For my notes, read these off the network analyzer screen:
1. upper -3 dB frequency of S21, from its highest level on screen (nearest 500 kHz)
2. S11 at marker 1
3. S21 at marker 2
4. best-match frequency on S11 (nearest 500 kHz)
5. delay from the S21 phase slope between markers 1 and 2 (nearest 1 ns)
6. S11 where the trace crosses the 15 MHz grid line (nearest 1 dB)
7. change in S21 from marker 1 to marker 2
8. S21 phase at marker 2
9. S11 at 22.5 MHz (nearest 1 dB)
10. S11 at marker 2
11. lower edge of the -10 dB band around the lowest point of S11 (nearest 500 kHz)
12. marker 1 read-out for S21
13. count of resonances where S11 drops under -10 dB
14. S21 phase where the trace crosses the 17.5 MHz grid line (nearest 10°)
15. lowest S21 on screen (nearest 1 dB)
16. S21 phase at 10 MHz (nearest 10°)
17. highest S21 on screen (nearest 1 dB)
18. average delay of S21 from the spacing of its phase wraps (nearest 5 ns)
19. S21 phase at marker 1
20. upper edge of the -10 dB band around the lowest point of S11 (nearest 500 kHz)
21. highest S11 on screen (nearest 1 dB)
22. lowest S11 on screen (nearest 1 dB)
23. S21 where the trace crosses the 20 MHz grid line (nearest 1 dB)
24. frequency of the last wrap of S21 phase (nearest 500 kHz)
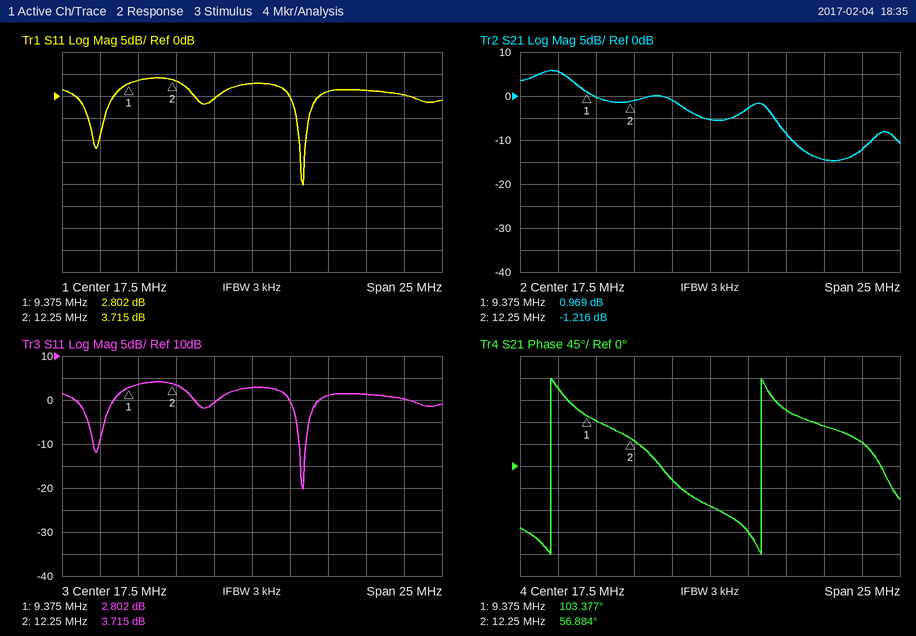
8.5 MHz
2.802 dB
-1.216 dB
21.0 MHz
45 ns
-1 dB
-2.185 dB
56.884°
1 dB
3.715 dB
20.5 MHz
0.969 dB
2
-80°
-15 dB
90°
6 dB
70 ns
103.377°
21.0 MHz
4 dB
-20 dB
-3 dB
21.0 MHz
